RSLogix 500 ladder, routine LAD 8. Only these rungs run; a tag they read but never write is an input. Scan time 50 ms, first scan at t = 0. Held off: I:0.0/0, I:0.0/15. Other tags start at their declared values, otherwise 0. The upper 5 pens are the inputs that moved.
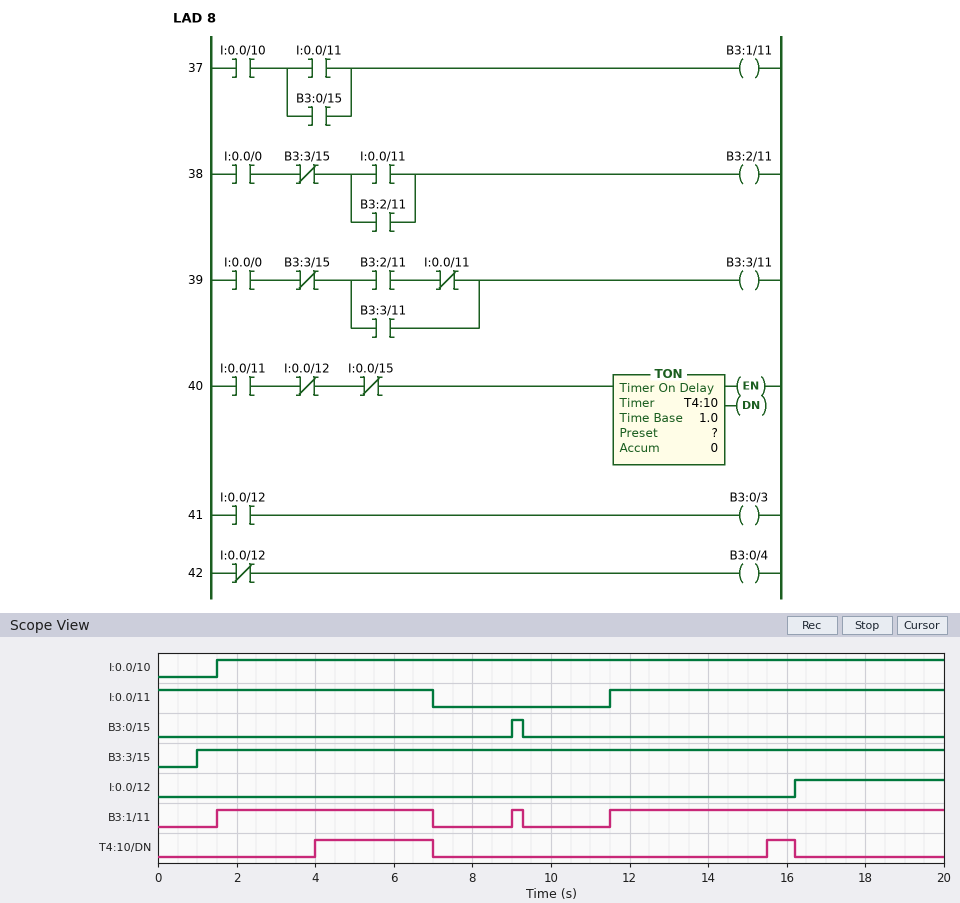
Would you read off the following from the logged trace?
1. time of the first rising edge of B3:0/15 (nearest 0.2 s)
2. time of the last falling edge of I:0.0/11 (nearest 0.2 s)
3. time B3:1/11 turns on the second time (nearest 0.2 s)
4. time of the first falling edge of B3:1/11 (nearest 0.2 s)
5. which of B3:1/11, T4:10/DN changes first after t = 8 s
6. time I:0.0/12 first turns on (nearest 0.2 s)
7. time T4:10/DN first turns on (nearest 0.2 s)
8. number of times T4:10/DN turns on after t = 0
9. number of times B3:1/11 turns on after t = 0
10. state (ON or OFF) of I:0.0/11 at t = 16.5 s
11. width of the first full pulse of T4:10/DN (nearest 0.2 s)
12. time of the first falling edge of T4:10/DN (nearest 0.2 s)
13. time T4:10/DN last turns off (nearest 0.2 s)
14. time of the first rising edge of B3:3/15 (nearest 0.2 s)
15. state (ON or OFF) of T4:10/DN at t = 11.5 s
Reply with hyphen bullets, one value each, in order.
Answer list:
- 9.0 s
- 7.0 s
- 9.0 s
- 7.0 s
- B3:1/11
- 16.2 s
- 4.0 s
- 2
- 3
- ON
- 3.0 s
- 7.0 s
- 16.2 s
- 1.0 s
- OFF
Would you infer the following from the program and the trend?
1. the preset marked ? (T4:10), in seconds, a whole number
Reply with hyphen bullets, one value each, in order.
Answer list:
- 4 s
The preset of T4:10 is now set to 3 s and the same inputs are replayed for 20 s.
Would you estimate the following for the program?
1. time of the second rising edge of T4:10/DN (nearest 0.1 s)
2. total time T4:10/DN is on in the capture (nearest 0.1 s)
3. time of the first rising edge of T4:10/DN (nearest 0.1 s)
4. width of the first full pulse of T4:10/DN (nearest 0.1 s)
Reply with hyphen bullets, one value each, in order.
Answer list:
- 14.5 s
- 5.7 s
- 3.0 s
- 4.0 s
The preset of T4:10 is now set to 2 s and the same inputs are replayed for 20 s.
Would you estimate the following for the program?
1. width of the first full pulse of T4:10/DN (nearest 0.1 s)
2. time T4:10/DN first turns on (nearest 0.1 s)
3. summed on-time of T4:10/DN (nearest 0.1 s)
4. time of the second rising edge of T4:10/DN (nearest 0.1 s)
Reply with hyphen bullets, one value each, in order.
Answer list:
- 5.0 s
- 2.0 s
- 7.7 s
- 13.5 s
